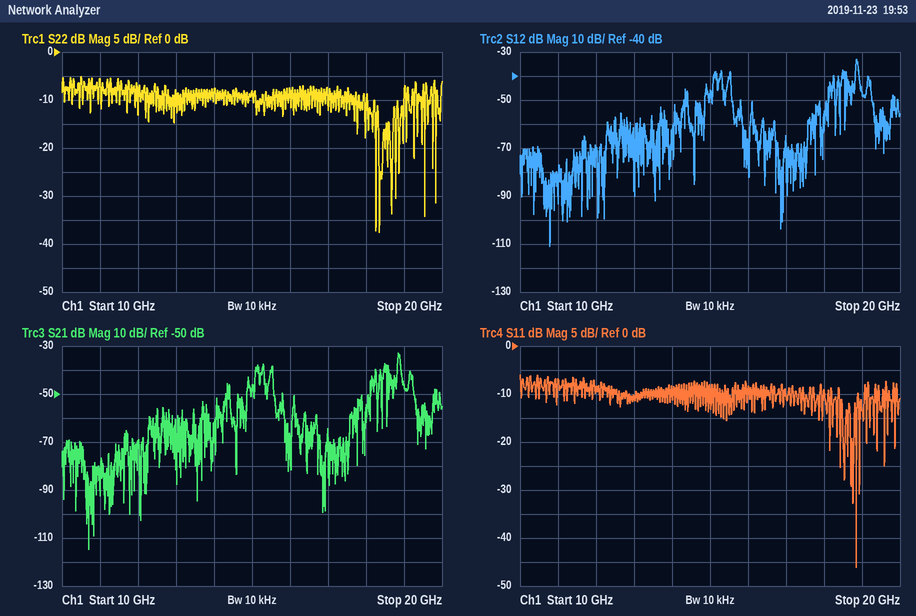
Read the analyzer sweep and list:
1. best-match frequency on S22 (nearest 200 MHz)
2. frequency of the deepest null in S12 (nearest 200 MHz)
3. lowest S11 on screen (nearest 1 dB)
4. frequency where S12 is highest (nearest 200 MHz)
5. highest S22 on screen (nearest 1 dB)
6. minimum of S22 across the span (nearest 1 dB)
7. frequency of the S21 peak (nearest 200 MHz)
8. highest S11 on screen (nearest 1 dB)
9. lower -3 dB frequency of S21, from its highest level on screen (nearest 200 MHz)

18.4 GHz
10.8 GHz
-46 dB
18.8 GHz
-5 dB
-38 dB
18.8 GHz
-6 dB
18.8 GHz
